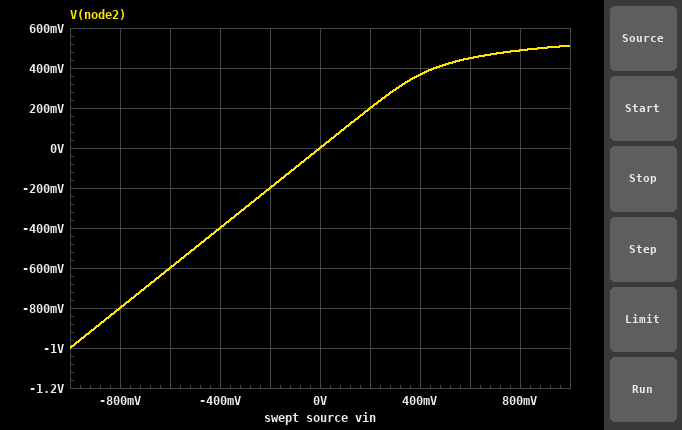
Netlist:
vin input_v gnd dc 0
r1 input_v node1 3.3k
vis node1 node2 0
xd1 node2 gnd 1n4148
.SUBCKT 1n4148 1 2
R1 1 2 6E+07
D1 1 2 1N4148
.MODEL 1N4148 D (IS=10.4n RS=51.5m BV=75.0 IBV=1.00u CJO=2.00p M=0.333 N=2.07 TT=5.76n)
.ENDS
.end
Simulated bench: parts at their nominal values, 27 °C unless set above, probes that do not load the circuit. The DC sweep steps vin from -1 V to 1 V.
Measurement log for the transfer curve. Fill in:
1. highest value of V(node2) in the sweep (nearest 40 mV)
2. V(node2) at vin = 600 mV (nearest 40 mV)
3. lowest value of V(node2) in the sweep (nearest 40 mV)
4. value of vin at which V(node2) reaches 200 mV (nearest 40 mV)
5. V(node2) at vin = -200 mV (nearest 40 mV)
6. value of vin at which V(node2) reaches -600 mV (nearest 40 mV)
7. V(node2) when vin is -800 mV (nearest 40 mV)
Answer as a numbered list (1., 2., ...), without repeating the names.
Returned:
1. 520 mV
2. 440 mV
3. -1.00 V
4. 200 mV
5. -200 mV
6. -600 mV
7. -800 mV
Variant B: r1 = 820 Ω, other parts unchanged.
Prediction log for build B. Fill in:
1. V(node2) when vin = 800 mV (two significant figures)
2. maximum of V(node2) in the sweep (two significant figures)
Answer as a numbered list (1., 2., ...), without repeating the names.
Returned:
1. 550 mV
2. 580 mV
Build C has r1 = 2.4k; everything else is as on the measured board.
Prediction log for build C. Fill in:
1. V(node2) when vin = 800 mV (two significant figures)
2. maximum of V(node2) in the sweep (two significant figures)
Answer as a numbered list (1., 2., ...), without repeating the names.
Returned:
1. 500 mV
2. 530 mV
